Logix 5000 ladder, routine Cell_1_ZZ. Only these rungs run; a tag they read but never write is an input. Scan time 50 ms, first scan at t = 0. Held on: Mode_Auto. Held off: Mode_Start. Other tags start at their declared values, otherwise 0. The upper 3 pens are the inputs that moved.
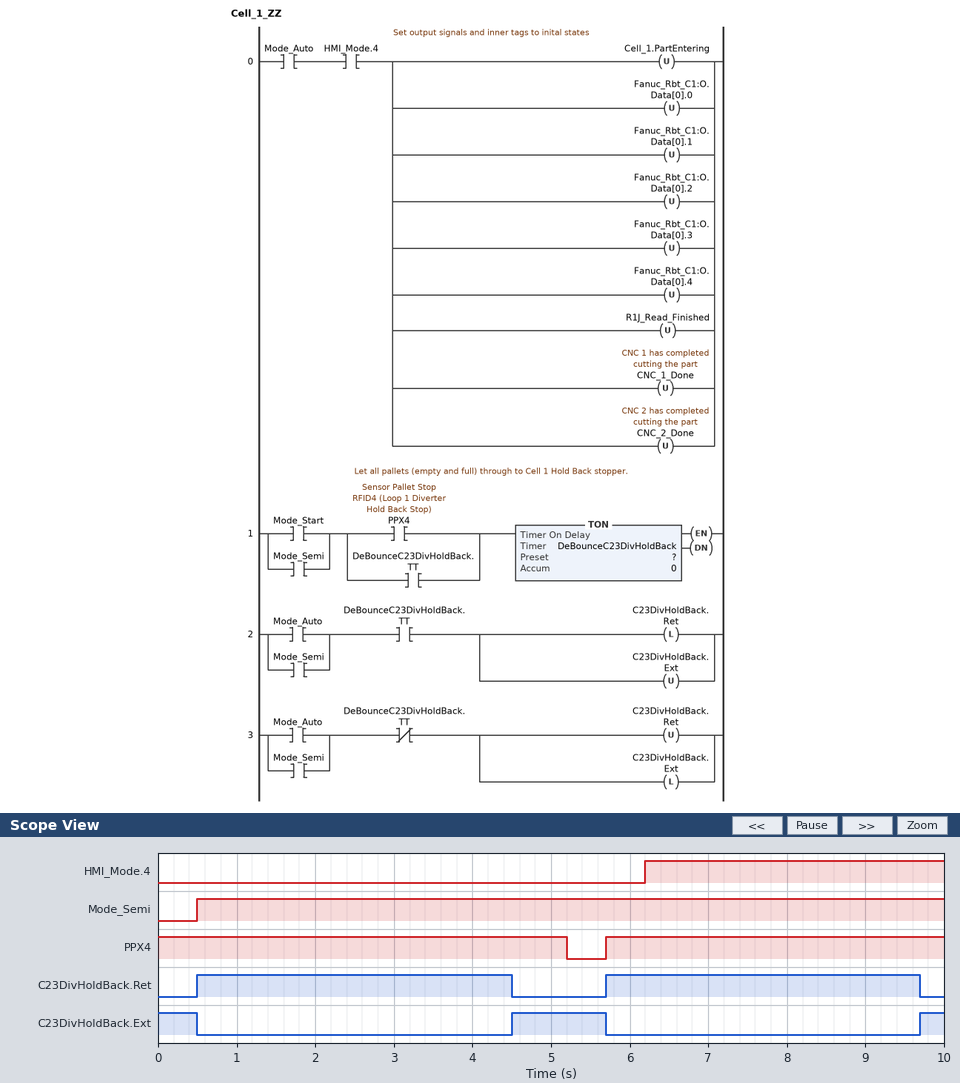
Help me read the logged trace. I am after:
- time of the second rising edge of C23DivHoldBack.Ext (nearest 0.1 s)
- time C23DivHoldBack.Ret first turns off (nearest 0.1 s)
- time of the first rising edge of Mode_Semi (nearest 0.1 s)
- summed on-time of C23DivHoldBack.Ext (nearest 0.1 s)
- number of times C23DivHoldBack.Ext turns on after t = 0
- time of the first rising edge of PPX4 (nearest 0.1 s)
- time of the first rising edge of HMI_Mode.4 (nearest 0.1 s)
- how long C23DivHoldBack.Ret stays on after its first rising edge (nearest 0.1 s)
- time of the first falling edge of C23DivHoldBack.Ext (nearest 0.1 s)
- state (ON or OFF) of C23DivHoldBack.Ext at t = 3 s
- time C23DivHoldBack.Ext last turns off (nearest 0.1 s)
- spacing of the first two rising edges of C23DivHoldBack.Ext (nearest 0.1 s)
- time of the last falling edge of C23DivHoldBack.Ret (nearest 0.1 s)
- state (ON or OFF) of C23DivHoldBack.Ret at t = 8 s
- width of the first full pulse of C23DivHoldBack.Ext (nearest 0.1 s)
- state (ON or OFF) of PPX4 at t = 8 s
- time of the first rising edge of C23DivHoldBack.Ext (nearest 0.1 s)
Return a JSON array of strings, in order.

["9.7 s", "4.5 s", "0.5 s", "2.0 s", "2", "5.7 s", "6.2 s", "4.0 s", "0.5 s", "OFF", "5.7 s", "5.2 s", "9.7 s", "ON", "1.2 s", "ON", "4.5 s"]
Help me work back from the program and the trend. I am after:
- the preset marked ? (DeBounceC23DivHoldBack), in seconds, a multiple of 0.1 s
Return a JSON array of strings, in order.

["4.0 s"]
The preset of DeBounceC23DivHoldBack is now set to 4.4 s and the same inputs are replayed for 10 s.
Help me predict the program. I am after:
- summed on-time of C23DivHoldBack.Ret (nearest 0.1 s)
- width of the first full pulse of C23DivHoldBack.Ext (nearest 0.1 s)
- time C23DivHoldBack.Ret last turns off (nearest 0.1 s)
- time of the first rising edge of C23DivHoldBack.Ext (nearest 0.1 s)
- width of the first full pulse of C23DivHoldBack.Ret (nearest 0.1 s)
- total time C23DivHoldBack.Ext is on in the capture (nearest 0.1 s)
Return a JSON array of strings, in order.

["8.7 s", "0.8 s", "4.9 s", "4.9 s", "4.4 s", "1.3 s"]
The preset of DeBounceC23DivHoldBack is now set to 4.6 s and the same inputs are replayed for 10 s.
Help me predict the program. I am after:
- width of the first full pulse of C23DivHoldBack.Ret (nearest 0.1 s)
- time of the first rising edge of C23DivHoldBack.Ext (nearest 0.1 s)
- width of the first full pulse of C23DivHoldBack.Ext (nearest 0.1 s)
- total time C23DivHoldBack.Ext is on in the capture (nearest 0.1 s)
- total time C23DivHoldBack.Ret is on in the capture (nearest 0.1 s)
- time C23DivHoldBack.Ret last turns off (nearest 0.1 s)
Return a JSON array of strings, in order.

["4.6 s", "5.1 s", "0.6 s", "1.1 s", "8.9 s", "5.1 s"]
